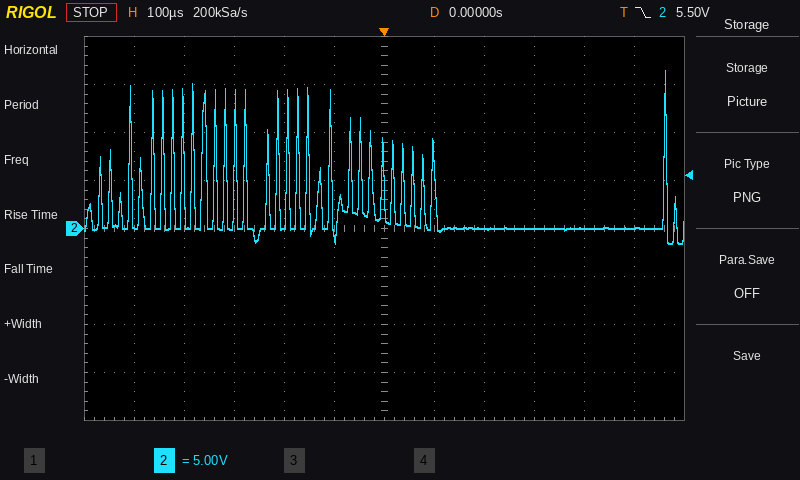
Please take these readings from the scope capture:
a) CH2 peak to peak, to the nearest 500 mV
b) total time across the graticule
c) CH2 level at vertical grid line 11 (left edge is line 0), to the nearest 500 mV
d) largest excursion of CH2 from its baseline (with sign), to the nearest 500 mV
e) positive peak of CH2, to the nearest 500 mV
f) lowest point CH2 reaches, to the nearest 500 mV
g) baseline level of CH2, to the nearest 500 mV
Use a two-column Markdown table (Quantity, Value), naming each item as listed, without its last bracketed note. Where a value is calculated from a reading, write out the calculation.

| Quantity | Value |
|---|---|
| CH2 peak to peak, to the nearest 500 mV | 16.5 V − (-1.5 V) = 18.0 V |
| total time across the graticule | 1.2 ms |
| CH2 level at vertical grid line 11 (left edge is line 0), to the nearest 500 mV | 0.0 V |
| largest excursion of CH2 from its baseline (with sign), to the nearest 500 mV | 16.5 V − (0.0 V) = +16.5 V |
| positive peak of CH2, to the nearest 500 mV | 16.5 V |
| lowest point CH2 reaches, to the nearest 500 mV | -1.5 V |
| baseline level of CH2, to the nearest 500 mV | 0.0 V |
